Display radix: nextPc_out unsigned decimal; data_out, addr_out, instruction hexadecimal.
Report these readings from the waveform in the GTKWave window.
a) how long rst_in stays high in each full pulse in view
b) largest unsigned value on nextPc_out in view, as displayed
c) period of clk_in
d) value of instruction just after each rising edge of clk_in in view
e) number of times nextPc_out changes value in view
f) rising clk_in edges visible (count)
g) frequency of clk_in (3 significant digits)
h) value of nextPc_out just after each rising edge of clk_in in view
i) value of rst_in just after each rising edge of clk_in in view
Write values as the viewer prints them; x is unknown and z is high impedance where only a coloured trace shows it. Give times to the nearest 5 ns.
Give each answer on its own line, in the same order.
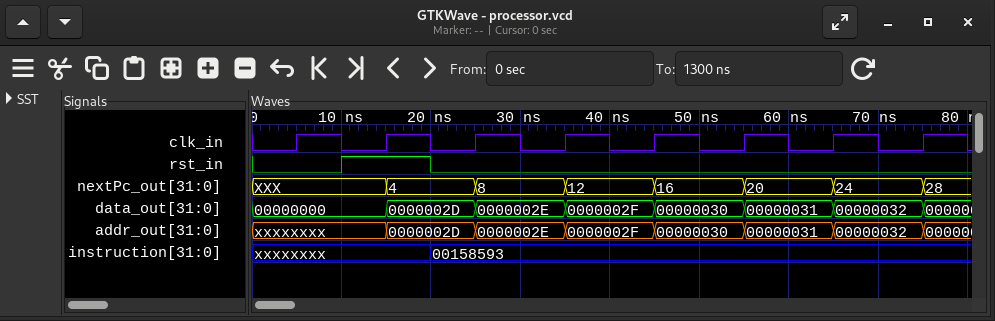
10 ns
28
10 ns
xxxxxxxx, xxxxxxxx, 00158593, 00158593, 00158593, 00158593, 00158593, 00158593
7
8
100 MHz
XXX, 4, 8, 12, 16, 20, 24, 28
0 1 0 0 0 0 0 0
